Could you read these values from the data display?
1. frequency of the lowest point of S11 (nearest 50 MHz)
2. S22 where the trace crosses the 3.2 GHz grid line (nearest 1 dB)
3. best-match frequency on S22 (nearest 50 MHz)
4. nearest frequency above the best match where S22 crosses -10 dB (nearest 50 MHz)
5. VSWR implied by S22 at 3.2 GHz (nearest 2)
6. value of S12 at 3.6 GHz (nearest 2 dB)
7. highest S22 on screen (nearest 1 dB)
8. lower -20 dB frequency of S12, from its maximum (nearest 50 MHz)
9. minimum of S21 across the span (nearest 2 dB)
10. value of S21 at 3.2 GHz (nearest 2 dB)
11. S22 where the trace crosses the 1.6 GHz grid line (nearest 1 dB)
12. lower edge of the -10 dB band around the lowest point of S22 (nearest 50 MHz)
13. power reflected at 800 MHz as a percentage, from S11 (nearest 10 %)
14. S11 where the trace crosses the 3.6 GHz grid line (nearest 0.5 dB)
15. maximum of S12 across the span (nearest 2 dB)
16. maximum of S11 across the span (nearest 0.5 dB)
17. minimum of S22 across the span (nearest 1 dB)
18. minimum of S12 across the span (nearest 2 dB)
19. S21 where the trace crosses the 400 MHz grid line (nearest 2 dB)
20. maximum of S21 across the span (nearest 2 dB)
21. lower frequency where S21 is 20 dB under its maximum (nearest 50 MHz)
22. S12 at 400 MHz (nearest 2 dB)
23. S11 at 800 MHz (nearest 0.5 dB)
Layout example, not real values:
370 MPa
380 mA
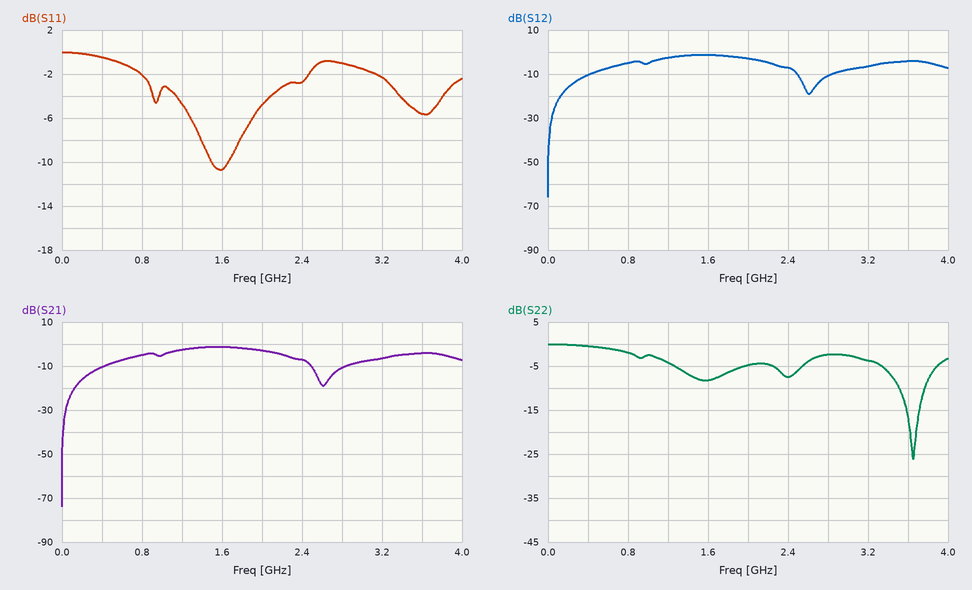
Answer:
1.60 GHz
-4 dB
3.65 GHz
3.75 GHz
4
-4 dB
0 dB
100 MHz
-74 dB
-6 dB
-8 dB
3.50 GHz
60 %
-5.5 dB
-2 dB
0.0 dB
-26 dB
-66 dB
-10 dB
-2 dB
100 MHz
-10 dB
-2.0 dB
